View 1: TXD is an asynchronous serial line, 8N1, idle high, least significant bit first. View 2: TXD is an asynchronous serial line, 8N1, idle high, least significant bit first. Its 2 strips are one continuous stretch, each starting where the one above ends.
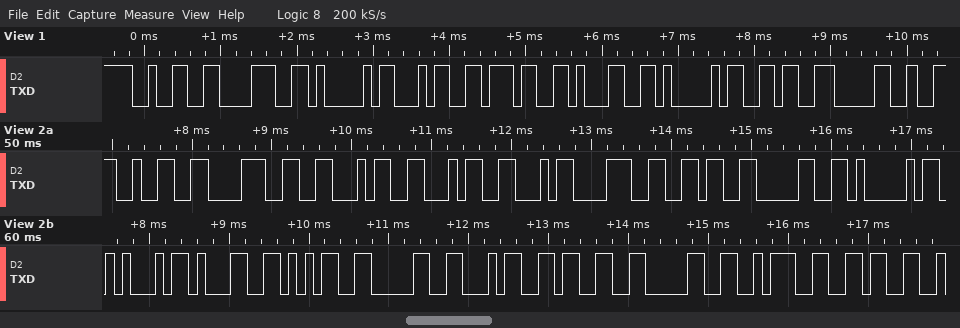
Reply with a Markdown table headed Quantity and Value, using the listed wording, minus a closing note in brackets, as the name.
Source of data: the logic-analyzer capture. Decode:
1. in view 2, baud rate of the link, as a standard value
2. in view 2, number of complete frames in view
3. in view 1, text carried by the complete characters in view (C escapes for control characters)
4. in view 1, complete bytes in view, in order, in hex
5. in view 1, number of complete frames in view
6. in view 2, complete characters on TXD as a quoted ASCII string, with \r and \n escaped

| Quantity | Value |
|---|---|
| in view 2, baud rate of the link, as a standard value | 9600 baud |
| in view 2, number of complete frames in view | 18 |
| in view 1, text carried by the complete characters in view | "28A471A60" |
| in view 1, complete bytes in view, in order, in hex | 32 38 41 34 37 31 41 36 30 |
| in view 1, number of complete frames in view | 9 |
| in view 2, complete characters on TXD as a quoted ASCII string, with \r and \n escaped | "28FFF860AE150430:6" |
